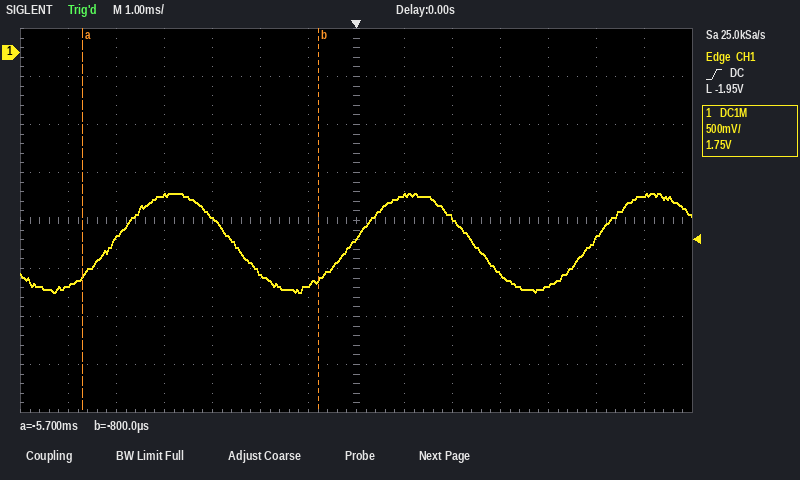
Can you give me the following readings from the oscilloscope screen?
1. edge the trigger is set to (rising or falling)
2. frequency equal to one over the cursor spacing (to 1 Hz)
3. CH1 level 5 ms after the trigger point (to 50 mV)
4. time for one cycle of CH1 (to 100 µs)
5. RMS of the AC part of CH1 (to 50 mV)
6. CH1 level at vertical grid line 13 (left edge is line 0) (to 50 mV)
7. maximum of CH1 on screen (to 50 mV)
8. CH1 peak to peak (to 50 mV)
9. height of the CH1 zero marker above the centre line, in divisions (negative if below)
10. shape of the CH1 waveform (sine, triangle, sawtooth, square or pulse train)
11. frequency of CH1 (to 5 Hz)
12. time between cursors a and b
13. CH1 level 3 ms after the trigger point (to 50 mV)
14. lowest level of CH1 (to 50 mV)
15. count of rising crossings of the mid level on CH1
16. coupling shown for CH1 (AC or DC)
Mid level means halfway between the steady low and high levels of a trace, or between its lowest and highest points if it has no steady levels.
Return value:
rising
204 Hz
-1.95 V
5.0 ms
350 mV
-1.50 V
-1.45 V
1.05 V
+3.5 div
sine
200 Hz
4.9 ms
-2.30 V
-2.50 V
3
DC
